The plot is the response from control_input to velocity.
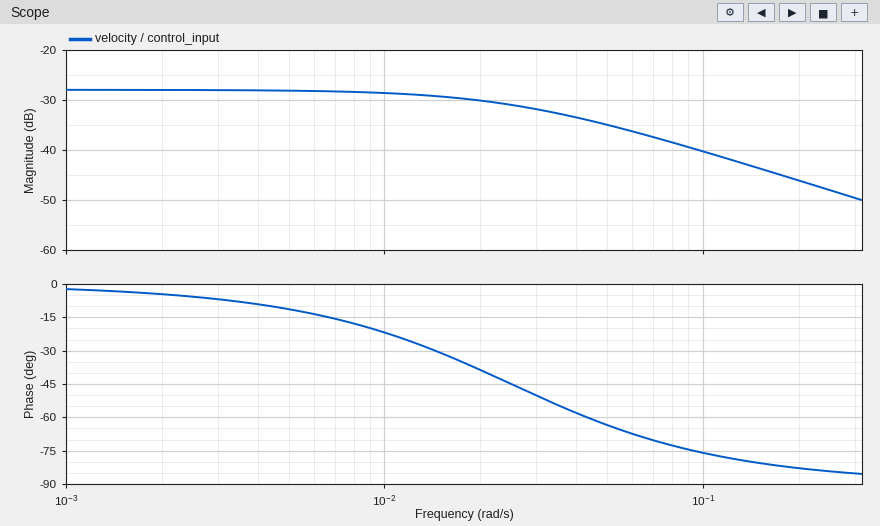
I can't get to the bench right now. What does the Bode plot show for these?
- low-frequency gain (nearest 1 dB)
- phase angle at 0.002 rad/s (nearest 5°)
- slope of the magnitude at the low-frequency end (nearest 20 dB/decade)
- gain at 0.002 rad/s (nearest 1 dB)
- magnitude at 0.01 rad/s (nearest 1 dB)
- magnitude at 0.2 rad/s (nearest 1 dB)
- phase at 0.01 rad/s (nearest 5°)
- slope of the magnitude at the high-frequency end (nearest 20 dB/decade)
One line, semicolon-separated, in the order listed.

-28 dB; -5°; 0 dB/decade; -28 dB; -29 dB; -46 dB; -20°; -20 dB/decade
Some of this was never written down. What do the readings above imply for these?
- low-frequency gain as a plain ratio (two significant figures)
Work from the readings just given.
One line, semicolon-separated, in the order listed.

0.040
